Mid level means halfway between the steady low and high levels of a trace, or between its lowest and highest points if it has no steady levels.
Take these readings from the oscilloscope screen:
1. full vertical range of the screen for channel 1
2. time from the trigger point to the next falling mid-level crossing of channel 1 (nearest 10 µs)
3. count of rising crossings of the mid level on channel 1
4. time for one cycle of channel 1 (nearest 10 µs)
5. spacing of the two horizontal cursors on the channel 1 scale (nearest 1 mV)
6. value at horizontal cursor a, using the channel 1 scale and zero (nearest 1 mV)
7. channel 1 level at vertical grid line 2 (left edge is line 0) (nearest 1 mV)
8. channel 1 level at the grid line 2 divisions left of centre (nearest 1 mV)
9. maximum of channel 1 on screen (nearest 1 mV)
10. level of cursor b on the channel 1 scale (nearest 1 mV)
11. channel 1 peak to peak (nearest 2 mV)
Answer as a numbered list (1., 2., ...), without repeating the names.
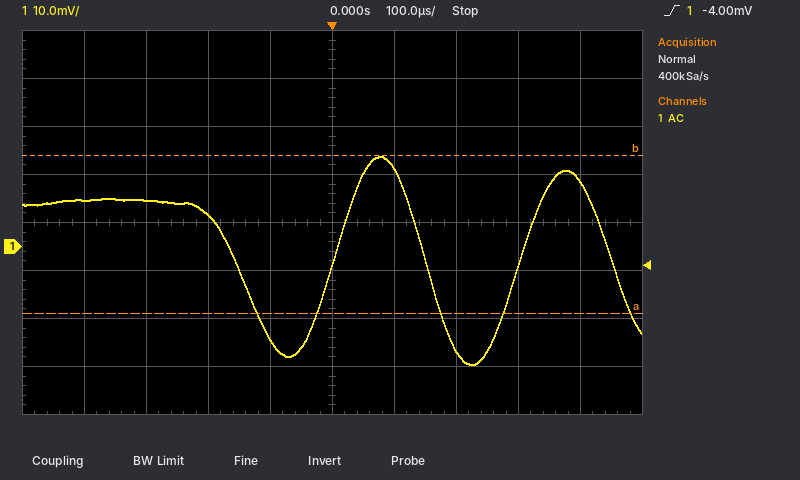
1. 80 mV
2. 150 µs
3. 2
4. 300 µs
5. 33 mV
6. -14 mV
7. 10 mV
8. 7 mV
9. 19 mV
10. 19 mV
11. 44 mV
